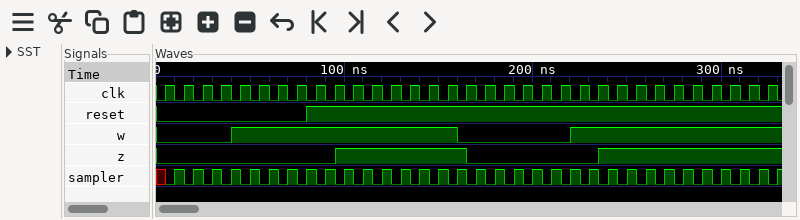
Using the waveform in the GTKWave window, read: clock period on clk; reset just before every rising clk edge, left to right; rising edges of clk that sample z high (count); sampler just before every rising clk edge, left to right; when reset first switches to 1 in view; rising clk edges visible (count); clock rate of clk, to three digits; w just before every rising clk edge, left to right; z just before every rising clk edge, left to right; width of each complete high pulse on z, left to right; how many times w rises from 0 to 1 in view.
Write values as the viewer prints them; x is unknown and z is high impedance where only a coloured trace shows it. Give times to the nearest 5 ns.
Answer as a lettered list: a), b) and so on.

a) 10 ns
b) 0 0 0 0 0 0 0 0 1 1 1 1 1 1 1 1 1 1 1 1 1 1 1 1 1 1 1 1 1 1 1 1 1
c) 16
d) x 1 1 1 1 1 1 1 1 1 1 1 1 1 1 1 1 1 1 1 1 1 1 1 1 1 1 1 1 1 1 1 1
e) 80 ns
f) 33
g) 100 MHz
h) 0 0 0 0 1 1 1 1 1 1 1 1 1 1 1 1 0 0 0 0 0 0 1 1 1 1 1 1 1 1 1 1 1
i) 0 0 0 0 0 0 0 0 0 0 1 1 1 1 1 1 1 0 0 0 0 0 0 0 1 1 1 1 1 1 1 1 1
j) 70 ns
k) 2
